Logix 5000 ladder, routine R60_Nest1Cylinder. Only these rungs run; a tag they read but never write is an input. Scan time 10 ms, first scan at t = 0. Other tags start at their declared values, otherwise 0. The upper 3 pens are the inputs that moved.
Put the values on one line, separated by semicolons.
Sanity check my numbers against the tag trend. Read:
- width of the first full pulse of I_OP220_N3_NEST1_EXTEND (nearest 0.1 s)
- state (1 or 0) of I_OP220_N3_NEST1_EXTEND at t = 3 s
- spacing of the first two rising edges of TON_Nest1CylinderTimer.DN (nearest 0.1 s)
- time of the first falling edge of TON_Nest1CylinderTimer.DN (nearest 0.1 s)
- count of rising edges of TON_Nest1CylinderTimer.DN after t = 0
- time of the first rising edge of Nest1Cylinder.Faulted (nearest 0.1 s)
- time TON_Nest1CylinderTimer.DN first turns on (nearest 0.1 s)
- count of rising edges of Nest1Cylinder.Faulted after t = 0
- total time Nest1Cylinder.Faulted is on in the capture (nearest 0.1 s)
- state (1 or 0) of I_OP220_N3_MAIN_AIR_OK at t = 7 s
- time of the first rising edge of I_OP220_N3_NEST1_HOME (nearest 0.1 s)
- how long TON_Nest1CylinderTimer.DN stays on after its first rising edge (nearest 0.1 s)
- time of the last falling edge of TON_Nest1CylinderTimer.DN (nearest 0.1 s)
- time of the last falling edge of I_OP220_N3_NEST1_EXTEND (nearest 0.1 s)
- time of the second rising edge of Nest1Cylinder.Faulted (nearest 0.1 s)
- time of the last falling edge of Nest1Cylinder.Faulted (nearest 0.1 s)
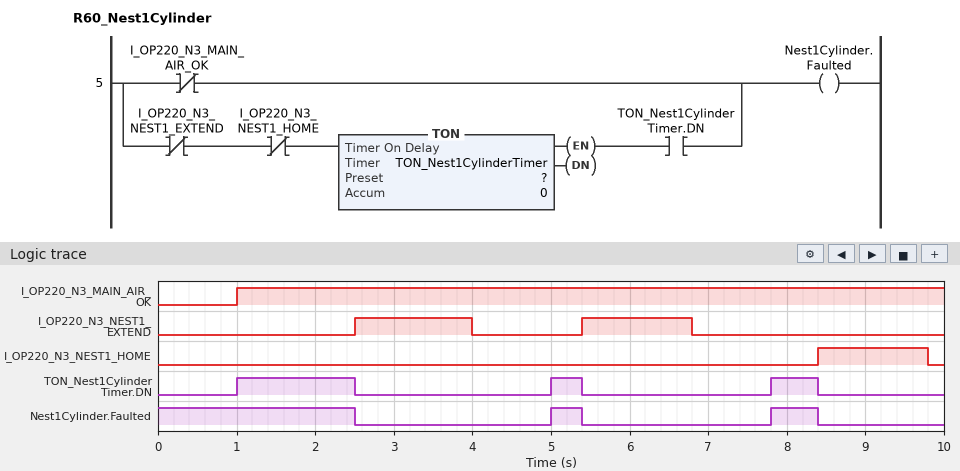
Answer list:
1.5 s; 1; 4.0 s; 2.5 s; 3; 5.0 s; 1.0 s; 2; 3.5 s; 1; 8.4 s; 1.5 s; 8.4 s; 6.8 s; 7.8 s; 8.4 s
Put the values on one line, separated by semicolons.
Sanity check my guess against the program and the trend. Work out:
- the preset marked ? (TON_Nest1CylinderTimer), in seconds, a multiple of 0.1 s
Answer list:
1.0 s
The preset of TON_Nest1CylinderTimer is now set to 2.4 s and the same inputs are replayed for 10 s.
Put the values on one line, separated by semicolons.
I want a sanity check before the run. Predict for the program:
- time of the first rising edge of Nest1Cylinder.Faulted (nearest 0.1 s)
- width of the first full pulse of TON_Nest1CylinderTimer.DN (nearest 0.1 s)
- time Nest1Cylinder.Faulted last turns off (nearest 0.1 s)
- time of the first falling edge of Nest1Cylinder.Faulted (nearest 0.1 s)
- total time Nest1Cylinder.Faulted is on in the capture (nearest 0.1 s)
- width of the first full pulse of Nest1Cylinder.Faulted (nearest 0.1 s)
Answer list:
2.4 s; 0.1 s; 2.5 s; 1.0 s; 1.1 s; 0.1 s
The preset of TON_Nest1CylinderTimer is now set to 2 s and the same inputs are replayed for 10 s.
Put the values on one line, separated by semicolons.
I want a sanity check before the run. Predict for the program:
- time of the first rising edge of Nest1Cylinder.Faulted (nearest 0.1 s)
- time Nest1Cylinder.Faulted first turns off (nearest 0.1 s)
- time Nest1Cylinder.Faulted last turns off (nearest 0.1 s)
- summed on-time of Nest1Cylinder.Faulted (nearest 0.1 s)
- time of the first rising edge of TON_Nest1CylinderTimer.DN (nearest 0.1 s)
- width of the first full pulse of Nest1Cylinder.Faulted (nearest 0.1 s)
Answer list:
2.0 s; 1.0 s; 2.5 s; 1.5 s; 2.0 s; 0.5 s
